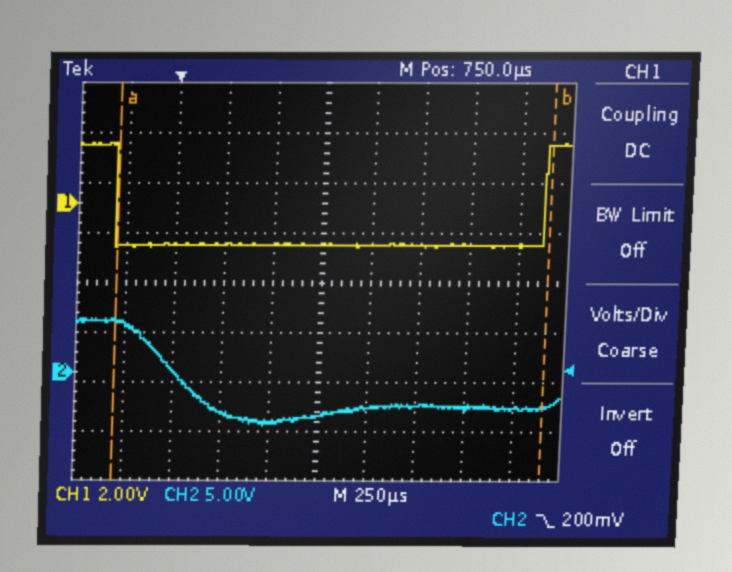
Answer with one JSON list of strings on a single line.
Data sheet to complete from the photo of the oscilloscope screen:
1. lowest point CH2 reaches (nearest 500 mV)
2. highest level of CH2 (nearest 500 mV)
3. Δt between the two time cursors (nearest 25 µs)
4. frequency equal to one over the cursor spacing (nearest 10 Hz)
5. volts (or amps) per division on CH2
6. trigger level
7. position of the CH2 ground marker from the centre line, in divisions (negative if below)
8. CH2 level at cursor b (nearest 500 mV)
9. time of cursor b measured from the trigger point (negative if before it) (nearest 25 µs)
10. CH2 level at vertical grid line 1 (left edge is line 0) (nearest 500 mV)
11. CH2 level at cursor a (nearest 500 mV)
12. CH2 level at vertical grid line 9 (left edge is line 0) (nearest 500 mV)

["-5.5 V", "5.5 V", "2.200 ms", "450 Hz", "5 V", "200 mV", "-1.8 div", "-3.5 V", "+1.900 ms", "5.0 V", "5.0 V", "-3.5 V"]
